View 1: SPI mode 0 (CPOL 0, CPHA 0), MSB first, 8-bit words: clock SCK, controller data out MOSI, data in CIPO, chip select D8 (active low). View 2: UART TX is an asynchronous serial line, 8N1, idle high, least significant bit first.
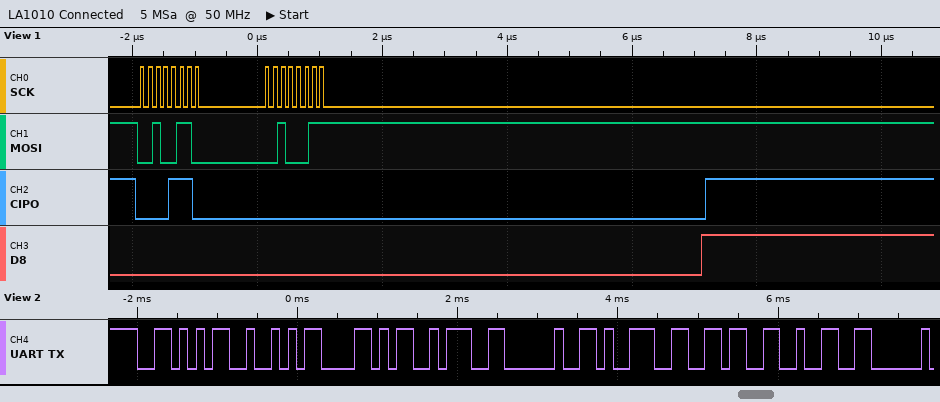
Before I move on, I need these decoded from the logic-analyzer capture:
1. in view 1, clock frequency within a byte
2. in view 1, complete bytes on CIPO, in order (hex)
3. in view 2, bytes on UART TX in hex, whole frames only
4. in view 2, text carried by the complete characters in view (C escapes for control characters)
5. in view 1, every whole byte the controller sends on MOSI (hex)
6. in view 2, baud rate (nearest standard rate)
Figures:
8 MHz
0E 00
56 52 58 3A 20 39 36 32
"VRX: 962"
26 23
9600 baud
